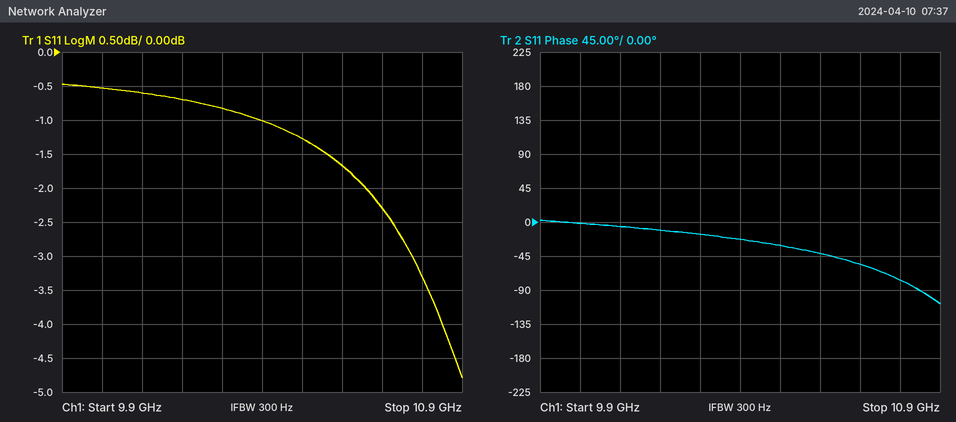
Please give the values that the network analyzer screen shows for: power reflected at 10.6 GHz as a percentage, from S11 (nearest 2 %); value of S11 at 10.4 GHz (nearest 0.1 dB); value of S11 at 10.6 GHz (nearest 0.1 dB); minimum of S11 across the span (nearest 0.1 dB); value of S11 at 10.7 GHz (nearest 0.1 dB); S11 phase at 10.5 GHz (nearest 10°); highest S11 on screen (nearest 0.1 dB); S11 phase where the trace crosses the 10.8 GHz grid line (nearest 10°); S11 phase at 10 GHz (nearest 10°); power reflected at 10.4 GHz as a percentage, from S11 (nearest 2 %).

68 %
-1.0 dB
-1.7 dB
-4.8 dB
-2.3 dB
-30°
-0.5 dB
-80°
0°
80 %
